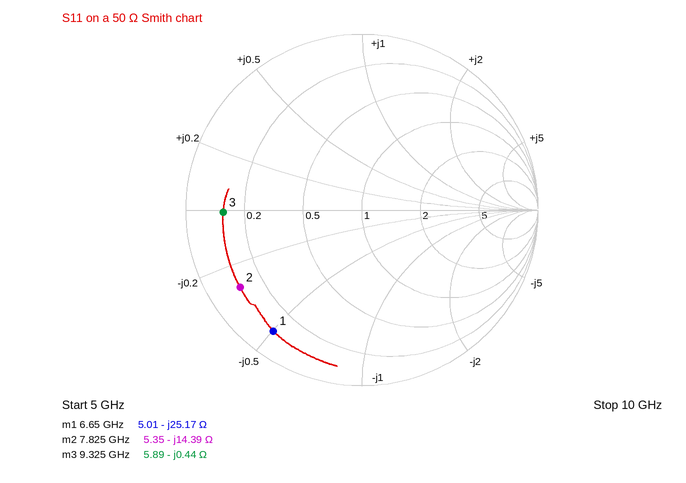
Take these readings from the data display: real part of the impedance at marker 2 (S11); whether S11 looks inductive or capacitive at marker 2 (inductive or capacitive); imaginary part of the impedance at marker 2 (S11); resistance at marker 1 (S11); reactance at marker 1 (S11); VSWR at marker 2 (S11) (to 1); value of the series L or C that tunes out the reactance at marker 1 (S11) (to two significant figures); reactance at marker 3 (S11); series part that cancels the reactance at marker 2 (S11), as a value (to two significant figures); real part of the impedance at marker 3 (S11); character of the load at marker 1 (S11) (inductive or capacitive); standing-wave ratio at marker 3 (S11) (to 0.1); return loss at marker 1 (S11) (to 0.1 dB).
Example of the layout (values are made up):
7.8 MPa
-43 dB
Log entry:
5.35 Ω
capacitive
-14.39 Ω
5.01 Ω
-25.17 Ω
10
600 pH
-0.44 Ω
290 pH
5.89 Ω
capacitive
8.5
1.4 dB
